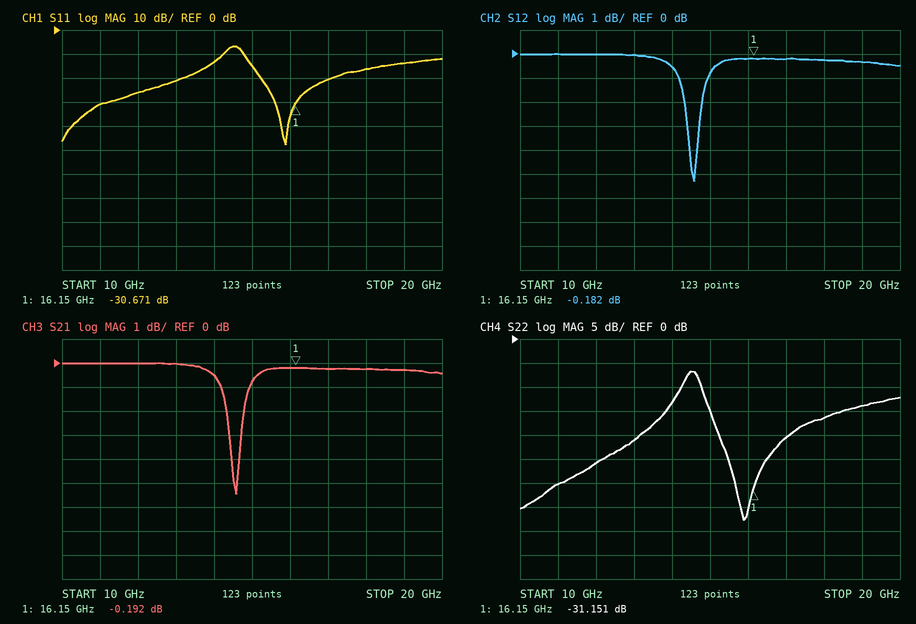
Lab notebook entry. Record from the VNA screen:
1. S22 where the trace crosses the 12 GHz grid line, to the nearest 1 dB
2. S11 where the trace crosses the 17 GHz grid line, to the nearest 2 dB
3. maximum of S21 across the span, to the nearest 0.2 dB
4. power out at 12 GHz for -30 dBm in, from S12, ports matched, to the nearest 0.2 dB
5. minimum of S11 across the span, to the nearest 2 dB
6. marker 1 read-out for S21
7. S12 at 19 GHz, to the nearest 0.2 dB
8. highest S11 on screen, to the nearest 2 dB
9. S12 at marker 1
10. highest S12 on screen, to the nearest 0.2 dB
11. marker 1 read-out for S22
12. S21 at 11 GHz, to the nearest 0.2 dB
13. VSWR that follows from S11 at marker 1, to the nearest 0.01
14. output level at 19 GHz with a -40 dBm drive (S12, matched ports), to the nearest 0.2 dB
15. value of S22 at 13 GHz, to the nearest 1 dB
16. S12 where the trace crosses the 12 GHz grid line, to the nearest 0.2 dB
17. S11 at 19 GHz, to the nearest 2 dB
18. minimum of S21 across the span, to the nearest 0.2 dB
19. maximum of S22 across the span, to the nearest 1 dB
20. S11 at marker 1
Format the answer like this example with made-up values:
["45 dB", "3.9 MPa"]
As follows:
["-26 dB", "-20 dB", "0.0 dB", "-30.0 dBm", "-48 dB", "-0.192 dB", "-0.4 dB", "-6 dB", "-0.182 dB", "0.0 dB", "-31.151 dB", "0.0 dB", "1.06", "-40.4 dBm", "-21 dB", "0.0 dB", "-14 dB", "-5.4 dB", "-7 dB", "-30.671 dB"]
